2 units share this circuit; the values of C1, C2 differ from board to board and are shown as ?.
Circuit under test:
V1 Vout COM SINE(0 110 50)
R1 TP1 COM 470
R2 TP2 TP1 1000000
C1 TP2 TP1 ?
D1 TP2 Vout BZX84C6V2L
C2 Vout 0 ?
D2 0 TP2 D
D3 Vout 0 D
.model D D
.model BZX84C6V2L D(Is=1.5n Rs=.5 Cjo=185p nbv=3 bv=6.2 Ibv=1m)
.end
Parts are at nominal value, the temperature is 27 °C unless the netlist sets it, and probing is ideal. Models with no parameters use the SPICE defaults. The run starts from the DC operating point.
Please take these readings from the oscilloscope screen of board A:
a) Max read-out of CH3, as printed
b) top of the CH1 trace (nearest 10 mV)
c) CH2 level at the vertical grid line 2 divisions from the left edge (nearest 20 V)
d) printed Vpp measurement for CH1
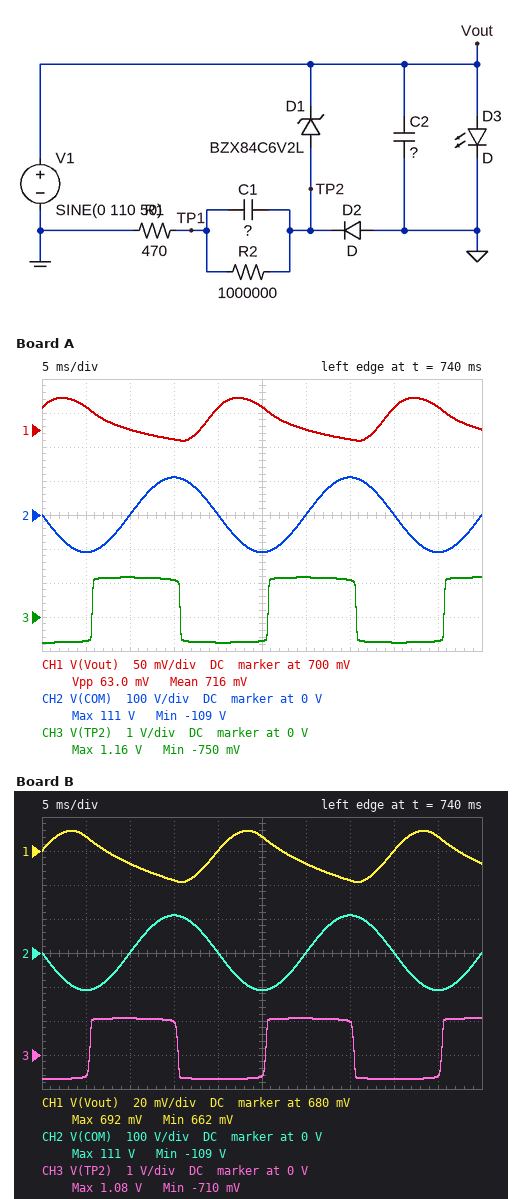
1.16 V
750 mV
0 V
63.0 mV
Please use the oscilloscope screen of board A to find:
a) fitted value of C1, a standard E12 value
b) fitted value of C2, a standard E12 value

1.2 µF
1.5 mF
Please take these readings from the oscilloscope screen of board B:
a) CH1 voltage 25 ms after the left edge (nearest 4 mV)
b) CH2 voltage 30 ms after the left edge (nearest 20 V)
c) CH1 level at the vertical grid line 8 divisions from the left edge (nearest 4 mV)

688 mV
0 V
680 mV
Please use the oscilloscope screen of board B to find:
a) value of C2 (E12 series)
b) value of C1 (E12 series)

820 µF
220 nF
